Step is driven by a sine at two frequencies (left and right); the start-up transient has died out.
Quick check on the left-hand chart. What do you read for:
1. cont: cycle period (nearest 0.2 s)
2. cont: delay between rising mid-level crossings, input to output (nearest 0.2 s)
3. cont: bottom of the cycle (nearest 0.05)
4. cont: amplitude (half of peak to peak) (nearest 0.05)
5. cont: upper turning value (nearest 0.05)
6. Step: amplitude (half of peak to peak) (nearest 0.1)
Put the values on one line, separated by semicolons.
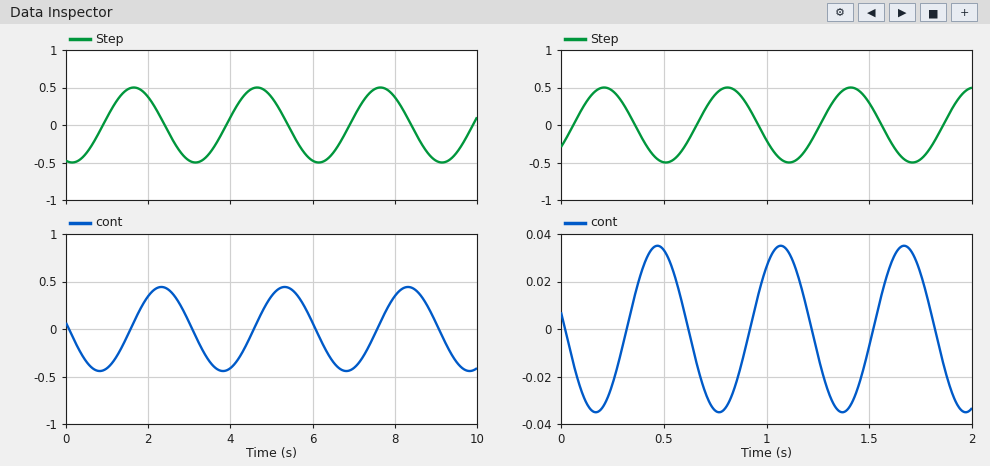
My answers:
3.0 s; 0.6 s; -0.45; 0.45; 0.45; 0.5
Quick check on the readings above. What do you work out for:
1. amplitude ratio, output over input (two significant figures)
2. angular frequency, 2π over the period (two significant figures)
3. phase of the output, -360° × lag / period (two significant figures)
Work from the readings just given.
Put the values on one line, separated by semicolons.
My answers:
0.90; 2.1 rad/s; -72°
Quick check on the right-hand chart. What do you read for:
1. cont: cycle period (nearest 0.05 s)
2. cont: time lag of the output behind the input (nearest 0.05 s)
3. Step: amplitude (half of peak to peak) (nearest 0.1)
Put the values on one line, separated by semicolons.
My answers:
0.60 s; 0.25 s; 0.5
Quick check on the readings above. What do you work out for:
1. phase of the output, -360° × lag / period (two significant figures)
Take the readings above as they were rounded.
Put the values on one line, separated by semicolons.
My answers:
-150°
